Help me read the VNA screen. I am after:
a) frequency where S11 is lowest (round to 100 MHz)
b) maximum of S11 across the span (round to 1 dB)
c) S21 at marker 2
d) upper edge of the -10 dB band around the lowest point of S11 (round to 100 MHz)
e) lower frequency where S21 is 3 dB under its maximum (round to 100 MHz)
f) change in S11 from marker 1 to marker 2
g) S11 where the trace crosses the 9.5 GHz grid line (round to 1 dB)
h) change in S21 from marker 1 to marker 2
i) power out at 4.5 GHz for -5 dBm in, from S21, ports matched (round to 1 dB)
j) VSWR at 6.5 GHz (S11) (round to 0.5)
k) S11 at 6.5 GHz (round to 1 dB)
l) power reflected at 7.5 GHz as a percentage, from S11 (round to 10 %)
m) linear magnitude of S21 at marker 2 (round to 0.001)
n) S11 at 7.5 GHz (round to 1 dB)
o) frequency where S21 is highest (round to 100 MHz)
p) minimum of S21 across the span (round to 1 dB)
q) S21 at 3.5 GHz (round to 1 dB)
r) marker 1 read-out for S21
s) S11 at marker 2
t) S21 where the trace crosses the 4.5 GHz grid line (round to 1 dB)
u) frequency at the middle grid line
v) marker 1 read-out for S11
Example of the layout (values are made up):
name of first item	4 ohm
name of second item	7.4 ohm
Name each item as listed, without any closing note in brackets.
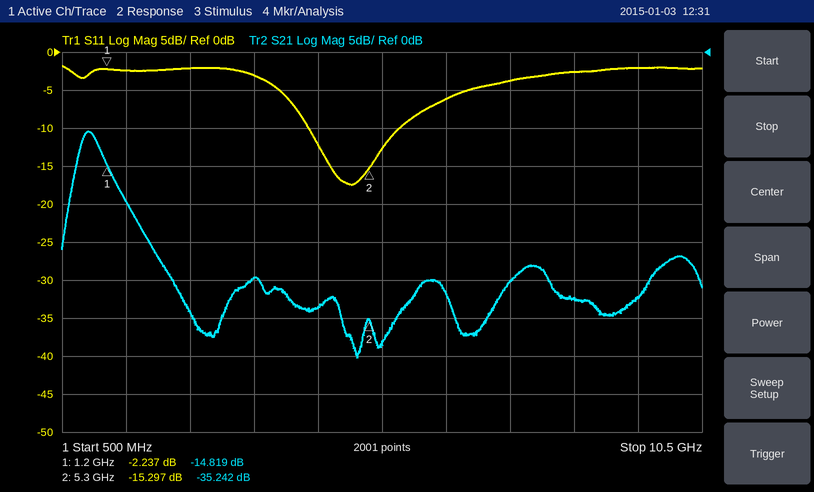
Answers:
frequency where S11 is lowest	5.0 GHz
maximum of S11 across the span	-2 dB
S21 at marker 2	-35.242 dB
upper edge of the -10 dB band around the lowest point of S11	5.8 GHz
lower frequency where S21 is 3 dB under its maximum	800 MHz
change in S11 from marker 1 to marker 2	-13.060 dB
S11 where the trace crosses the 9.5 GHz grid line	-2 dB
change in S21 from marker 1 to marker 2	-20.423 dB
power out at 4.5 GHz for -5 dBm in, from S21, ports matched	-39 dBm
VSWR at 6.5 GHz (S11)	3.0
S11 at 6.5 GHz	-6 dB
power reflected at 7.5 GHz as a percentage, from S11	40 %
linear magnitude of S21 at marker 2	0.017
S11 at 7.5 GHz	-4 dB
frequency where S21 is highest	900 MHz
minimum of S21 across the span	-40 dB
S21 at 3.5 GHz	-30 dB
marker 1 read-out for S21	-14.819 dB
S11 at marker 2	-15.297 dB
S21 where the trace crosses the 4.5 GHz grid line	-34 dB
frequency at the middle grid line	5.5 GHz
marker 1 read-out for S11	-2.237 dB
